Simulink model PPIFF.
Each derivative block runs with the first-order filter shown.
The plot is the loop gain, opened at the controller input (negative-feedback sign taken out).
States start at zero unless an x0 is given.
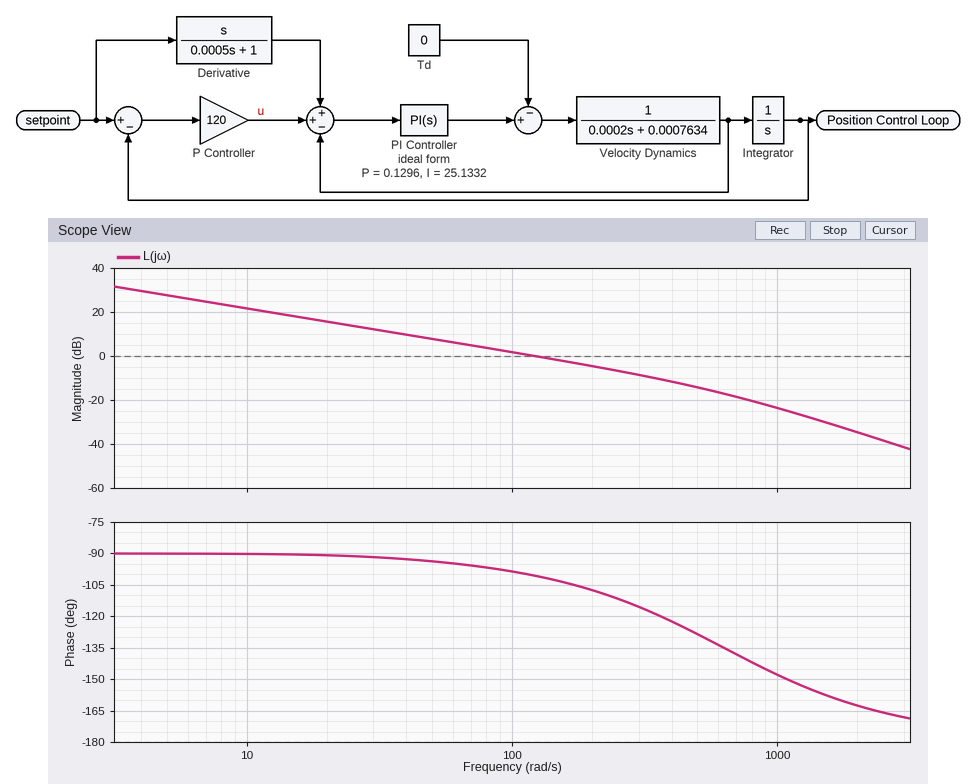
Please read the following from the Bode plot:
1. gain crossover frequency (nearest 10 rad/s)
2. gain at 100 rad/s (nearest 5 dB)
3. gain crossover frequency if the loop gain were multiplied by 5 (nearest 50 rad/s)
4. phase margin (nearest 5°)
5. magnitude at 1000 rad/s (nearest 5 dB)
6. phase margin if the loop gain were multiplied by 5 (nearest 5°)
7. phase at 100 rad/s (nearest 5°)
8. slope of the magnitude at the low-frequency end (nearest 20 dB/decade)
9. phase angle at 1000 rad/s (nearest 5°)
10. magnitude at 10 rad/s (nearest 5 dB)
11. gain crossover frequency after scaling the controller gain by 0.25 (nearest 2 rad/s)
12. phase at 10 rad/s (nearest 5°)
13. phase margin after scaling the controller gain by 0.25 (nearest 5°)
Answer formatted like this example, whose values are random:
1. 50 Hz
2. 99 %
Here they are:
1. 120 rad/s
2. 0 dB
3. 500 rad/s
4. 80°
5. -25 dB
6. 50°
7. -100°
8. -20 dB/decade
9. -150°
10. 20 dB
11. 30 rad/s
12. -90°
13. 90°
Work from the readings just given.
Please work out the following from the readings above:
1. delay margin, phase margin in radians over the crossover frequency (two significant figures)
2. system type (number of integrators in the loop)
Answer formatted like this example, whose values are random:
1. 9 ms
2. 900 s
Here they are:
1. 0.012 s
2. 1
